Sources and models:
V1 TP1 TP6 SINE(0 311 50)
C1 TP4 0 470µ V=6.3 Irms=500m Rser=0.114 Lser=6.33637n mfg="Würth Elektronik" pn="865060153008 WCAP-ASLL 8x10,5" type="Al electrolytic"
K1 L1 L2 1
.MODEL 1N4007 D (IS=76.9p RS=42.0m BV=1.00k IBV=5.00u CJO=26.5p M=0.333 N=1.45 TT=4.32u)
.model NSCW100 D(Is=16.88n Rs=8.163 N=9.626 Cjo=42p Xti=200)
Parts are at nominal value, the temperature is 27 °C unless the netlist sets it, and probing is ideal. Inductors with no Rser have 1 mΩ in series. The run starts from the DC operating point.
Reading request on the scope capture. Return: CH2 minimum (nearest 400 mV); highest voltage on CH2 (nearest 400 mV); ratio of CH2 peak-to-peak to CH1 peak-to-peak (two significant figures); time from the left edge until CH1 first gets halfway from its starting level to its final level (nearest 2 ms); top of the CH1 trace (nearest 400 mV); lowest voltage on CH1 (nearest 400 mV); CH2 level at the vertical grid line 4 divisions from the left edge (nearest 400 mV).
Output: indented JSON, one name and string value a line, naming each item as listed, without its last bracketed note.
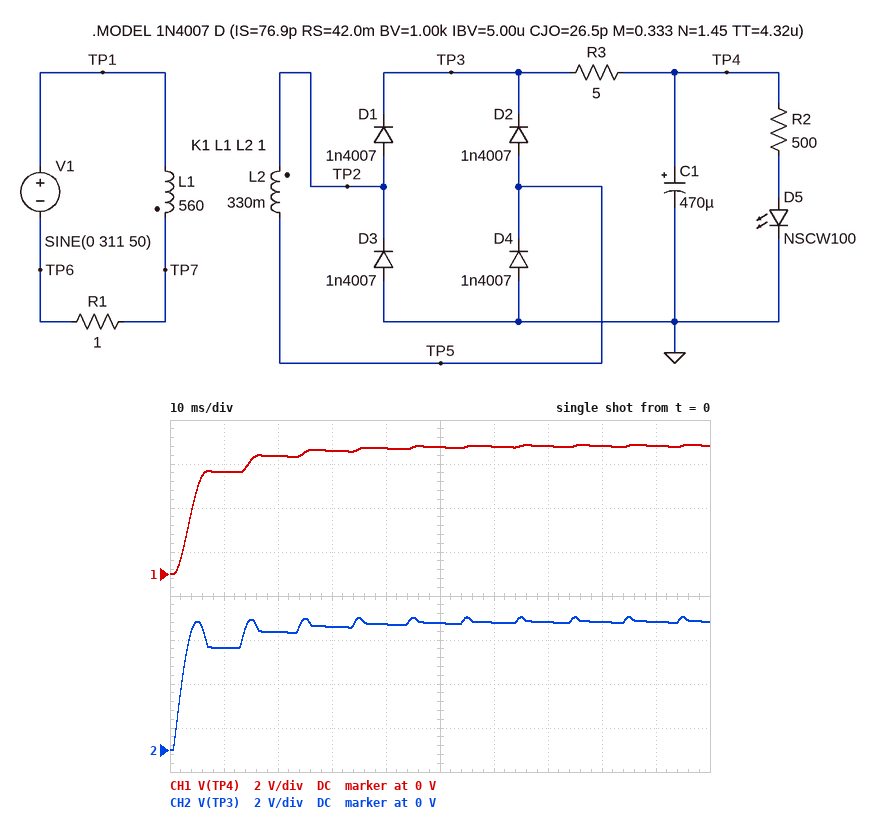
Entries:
{
  "CH2 minimum": "0 V",
  "highest voltage on CH2": "6.0 V",
  "ratio of CH2 peak-to-peak to CH1 peak-to-peak": "1.0",
  "time from the left edge until CH1 first gets halfway from its starting level to its final level": "4 ms",
  "top of the CH1 trace": "6.0 V",
  "lowest voltage on CH1": "0 V",
  "CH2 level at the vertical grid line 4 divisions from the left edge": "5.6 V"
}
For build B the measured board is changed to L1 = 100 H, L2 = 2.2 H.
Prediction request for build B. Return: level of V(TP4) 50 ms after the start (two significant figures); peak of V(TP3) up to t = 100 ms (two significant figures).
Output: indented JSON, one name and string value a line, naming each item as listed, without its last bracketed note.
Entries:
{
  "level of V(TP4) 50 ms after the start": "42 V",
  "peak of V(TP3) up to t = 100 ms": "44 V"
}
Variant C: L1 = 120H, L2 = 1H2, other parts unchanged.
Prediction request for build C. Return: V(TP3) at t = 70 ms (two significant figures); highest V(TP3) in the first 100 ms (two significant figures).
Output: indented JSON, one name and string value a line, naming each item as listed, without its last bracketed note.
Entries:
{
  "V(TP3) at t = 70 ms": "28 V",
  "highest V(TP3) in the first 100 ms": "29 V"
}
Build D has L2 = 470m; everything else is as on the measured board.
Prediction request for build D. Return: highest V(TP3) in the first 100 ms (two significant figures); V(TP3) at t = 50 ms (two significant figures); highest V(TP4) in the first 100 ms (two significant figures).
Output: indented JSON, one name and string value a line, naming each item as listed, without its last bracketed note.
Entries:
{
  "highest V(TP3) in the first 100 ms": "7.5 V",
  "V(TP3) at t = 50 ms": "7.1 V",
  "highest V(TP4) in the first 100 ms": "7.2 V"
}
